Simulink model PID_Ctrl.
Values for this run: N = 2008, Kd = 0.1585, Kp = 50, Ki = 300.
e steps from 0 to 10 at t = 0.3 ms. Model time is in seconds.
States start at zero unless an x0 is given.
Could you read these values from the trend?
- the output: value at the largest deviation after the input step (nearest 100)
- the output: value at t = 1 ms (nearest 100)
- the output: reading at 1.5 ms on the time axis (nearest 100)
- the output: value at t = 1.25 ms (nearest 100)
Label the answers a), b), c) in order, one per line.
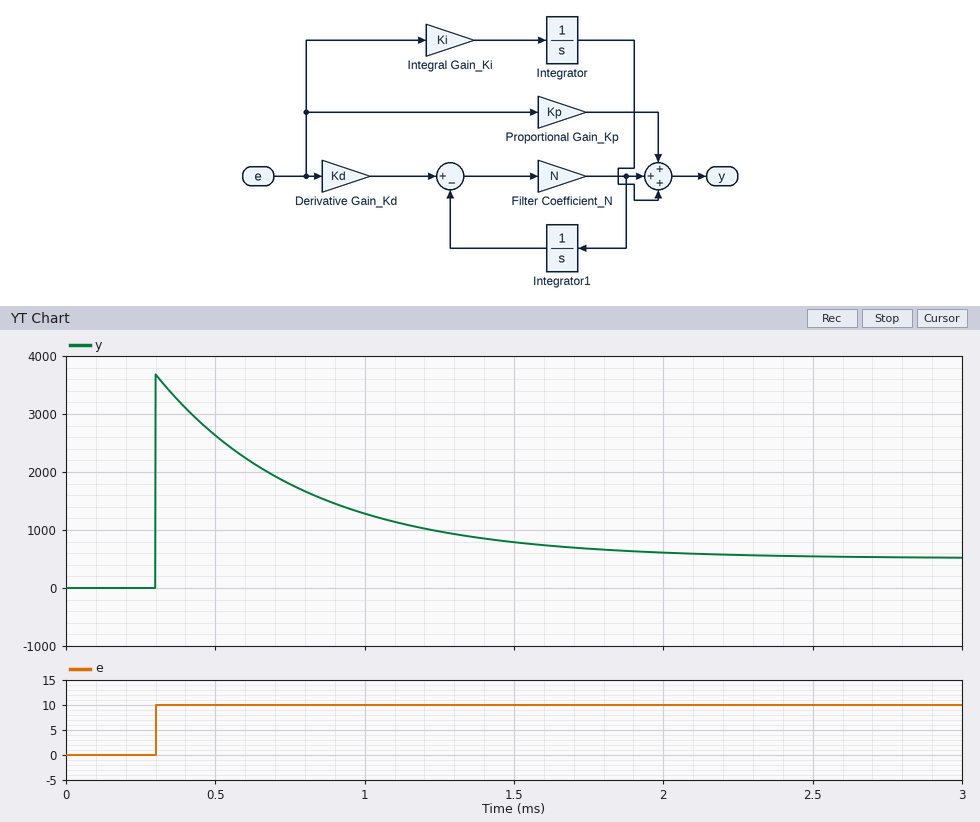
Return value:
a) 3700
b) 1300
c) 800
d) 1000
